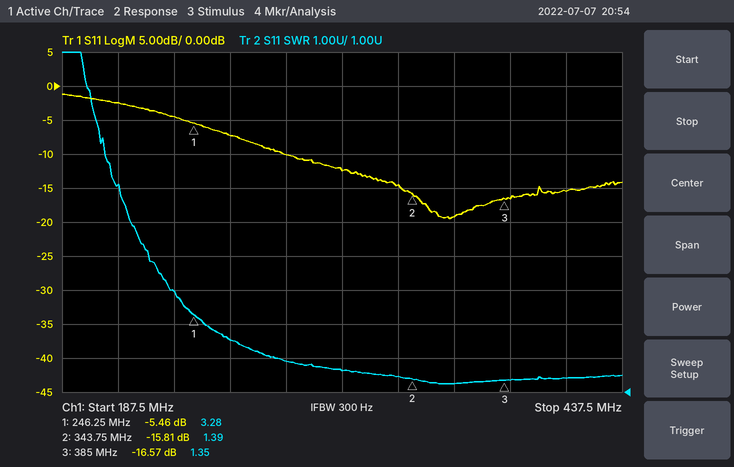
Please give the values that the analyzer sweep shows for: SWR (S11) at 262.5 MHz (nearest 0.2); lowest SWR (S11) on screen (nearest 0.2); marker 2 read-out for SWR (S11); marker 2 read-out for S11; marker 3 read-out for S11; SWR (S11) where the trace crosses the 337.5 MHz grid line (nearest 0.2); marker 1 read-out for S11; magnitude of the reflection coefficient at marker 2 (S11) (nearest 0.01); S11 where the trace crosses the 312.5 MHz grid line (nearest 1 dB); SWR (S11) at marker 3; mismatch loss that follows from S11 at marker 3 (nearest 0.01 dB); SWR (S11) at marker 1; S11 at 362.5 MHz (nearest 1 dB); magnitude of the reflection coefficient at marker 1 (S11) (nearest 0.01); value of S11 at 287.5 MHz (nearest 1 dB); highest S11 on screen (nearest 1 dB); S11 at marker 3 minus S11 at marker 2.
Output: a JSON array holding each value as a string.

["2.6", "1.2", "1.39", "-15.81 dB", "-16.57 dB", "1.4", "-5.46 dB", "0.16", "-12 dB", "1.35", "0.10 dB", "3.28", "-19 dB", "0.53", "-10 dB", "-1 dB", "-0.76 dB"]
